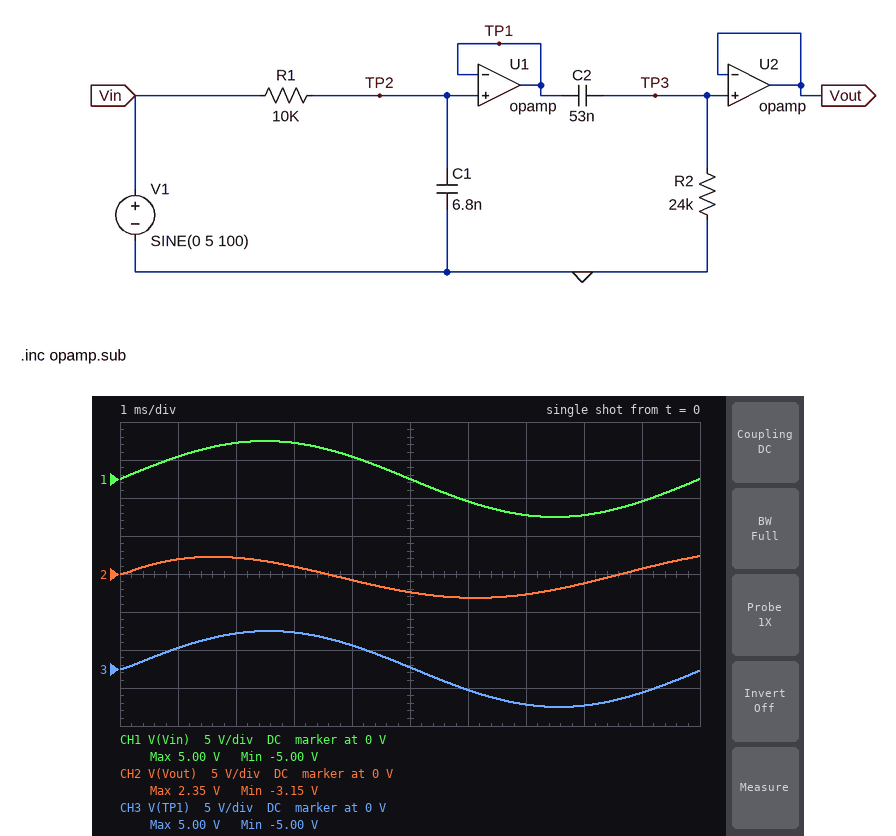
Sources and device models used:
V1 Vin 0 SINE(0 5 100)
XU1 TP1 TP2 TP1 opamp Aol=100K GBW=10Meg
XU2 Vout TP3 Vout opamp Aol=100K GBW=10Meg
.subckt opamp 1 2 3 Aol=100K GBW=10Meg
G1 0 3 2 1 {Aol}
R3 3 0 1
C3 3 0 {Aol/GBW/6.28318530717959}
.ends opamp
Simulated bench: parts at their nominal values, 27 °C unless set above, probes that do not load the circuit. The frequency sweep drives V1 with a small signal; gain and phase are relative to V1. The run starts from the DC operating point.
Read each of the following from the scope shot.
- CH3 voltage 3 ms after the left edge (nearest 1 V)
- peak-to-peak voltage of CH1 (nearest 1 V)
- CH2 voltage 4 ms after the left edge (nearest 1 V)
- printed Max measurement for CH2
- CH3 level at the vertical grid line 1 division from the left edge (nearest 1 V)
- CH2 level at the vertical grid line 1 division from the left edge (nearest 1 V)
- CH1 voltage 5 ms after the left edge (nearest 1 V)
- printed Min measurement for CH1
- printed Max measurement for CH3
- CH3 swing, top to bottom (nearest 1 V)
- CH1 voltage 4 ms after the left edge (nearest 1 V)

5 V
10 V
-1 V
2.35 V
3 V
2 V
0 V
-5.00 V
5.00 V
10 V
3 V
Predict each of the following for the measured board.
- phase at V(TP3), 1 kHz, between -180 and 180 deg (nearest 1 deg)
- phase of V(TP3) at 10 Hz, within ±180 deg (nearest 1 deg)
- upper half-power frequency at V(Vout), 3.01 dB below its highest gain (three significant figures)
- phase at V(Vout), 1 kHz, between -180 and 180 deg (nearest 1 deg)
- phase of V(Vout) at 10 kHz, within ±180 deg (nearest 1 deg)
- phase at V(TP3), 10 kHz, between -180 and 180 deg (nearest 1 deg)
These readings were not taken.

-16 deg
85 deg
2.58 kHz
-16 deg
-76 deg
-76 deg
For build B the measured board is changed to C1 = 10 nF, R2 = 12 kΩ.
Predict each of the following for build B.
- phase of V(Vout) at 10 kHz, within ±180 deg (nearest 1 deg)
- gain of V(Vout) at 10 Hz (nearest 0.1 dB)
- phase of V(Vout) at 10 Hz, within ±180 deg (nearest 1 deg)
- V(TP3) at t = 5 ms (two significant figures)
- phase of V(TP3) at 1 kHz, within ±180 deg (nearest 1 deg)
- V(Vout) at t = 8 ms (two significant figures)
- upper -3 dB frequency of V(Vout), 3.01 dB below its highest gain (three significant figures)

-80 deg
-28.0 dB
87 deg
-1.7 V
-18 deg
-240 mV
2.04 kHz
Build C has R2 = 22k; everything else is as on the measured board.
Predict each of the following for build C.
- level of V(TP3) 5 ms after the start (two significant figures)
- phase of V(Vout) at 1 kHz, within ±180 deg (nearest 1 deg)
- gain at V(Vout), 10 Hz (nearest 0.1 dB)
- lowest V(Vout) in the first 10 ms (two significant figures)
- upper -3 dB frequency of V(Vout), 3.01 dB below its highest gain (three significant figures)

-2.3 V
-15 deg
-22.7 dB
-3.0 V
2.60 kHz
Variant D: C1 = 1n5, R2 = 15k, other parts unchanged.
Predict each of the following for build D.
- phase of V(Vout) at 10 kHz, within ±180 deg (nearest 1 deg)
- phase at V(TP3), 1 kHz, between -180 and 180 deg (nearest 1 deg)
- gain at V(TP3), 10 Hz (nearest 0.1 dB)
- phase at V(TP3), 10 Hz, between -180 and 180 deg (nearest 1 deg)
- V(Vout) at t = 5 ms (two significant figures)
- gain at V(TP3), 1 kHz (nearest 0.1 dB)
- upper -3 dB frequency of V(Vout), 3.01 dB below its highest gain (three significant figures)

-42 deg
6 deg
-26.0 dB
87 deg
-2.0 V
-0.2 dB
11.0 kHz
